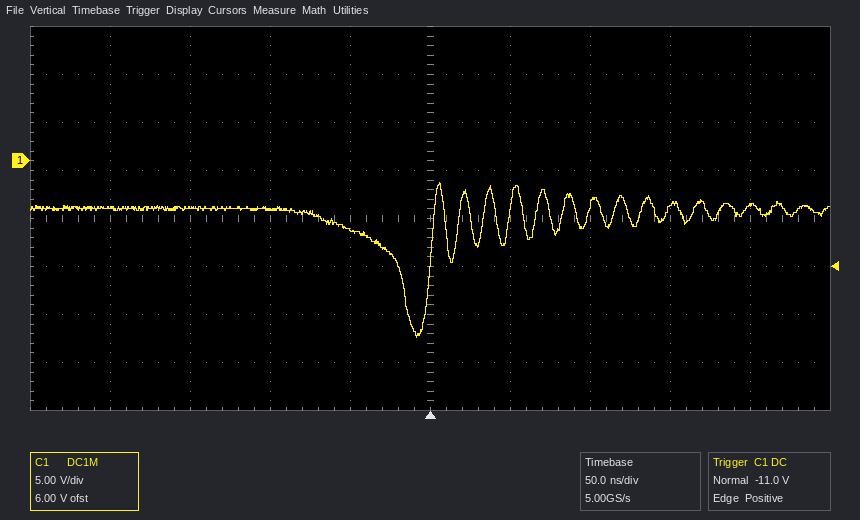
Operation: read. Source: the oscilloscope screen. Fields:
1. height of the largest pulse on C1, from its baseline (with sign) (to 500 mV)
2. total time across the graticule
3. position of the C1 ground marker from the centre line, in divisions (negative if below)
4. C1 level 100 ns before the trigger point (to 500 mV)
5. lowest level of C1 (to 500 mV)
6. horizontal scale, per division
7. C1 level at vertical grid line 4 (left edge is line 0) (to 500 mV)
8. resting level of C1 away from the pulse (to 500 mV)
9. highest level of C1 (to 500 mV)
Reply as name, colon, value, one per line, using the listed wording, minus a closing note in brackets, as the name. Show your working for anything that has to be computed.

height of the largest pulse on C1, from its baseline (with sign): -18.5 V − (-5.0 V) = -13.5 V
total time across the graticule: 500 ns
position of the C1 ground marker from the centre line, in divisions: +1.2 div
C1 level 100 ns before the trigger point: -5.0 V
lowest level of C1: -18.5 V
horizontal scale, per division: 50 ns
C1 level at vertical grid line 4 (left edge is line 0): -7.0 V
resting level of C1 away from the pulse: -5.0 V
highest level of C1: -2.0 V
